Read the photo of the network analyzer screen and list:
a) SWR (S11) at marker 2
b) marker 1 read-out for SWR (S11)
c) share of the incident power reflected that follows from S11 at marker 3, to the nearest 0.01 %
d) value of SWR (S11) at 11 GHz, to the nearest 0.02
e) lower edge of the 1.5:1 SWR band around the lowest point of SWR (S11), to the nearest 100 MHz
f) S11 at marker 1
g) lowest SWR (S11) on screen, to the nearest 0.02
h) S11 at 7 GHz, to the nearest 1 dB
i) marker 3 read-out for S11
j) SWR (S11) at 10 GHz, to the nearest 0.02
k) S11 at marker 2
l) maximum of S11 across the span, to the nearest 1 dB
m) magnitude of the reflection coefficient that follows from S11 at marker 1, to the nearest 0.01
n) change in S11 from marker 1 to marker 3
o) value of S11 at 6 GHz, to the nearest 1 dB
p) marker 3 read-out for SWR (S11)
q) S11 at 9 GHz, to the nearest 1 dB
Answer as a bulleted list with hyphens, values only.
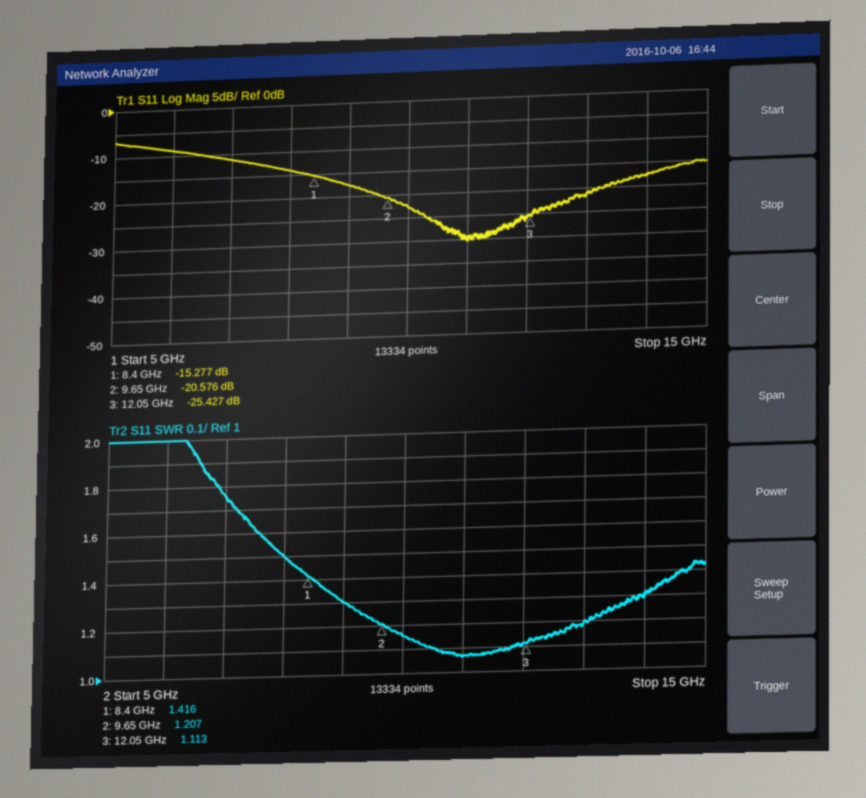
- 1.207
- 1.416
- 0.29 %
- 1.06
- 8.0 GHz
- -15.277 dB
- 1.06
- -11 dB
- -25.427 dB
- 1.16
- -20.576 dB
- -7 dB
- 0.17
- -10.150 dB
- -9 dB
- 1.113
- -18 dB
